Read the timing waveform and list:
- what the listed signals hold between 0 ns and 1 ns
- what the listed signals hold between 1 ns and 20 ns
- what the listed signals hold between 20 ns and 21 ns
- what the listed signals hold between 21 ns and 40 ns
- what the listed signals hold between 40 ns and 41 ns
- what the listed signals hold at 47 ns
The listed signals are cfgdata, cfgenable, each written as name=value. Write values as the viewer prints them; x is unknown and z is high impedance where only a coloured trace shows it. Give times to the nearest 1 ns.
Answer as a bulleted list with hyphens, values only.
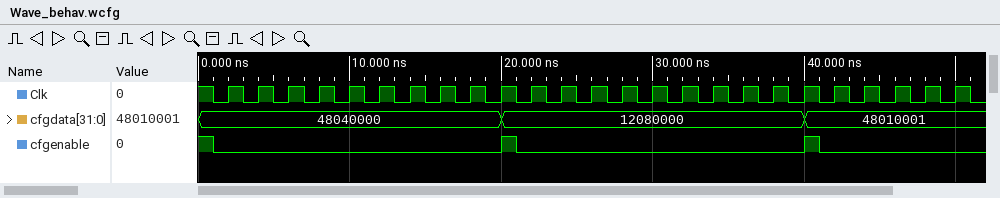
- cfgdata=48040000, cfgenable=1
- cfgdata=48040000, cfgenable=0
- cfgdata=12080000, cfgenable=1
- cfgdata=12080000, cfgenable=0
- cfgdata=48010001, cfgenable=1
- cfgdata=48010001, cfgenable=0
